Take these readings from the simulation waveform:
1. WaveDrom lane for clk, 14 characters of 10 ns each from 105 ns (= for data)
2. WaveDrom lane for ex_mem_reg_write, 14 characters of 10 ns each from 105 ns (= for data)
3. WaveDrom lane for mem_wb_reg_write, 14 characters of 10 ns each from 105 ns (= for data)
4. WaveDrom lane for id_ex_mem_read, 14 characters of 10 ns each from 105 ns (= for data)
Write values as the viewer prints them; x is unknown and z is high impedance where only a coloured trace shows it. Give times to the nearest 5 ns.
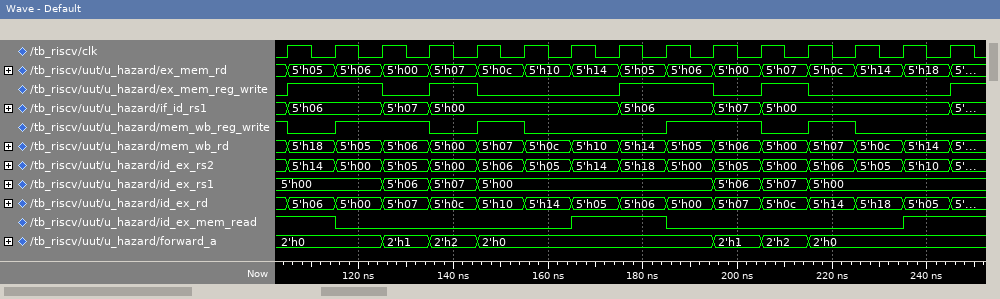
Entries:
{name: 'clk', wave: 'p.............'}
{name: 'ex_mem_reg_write', wave: '1.010..1.010..'}
{name: 'mem_wb_reg_write', wave: '01.010..1.010.'}
{name: 'id_ex_mem_read', wave: '10....1.0....1'}
